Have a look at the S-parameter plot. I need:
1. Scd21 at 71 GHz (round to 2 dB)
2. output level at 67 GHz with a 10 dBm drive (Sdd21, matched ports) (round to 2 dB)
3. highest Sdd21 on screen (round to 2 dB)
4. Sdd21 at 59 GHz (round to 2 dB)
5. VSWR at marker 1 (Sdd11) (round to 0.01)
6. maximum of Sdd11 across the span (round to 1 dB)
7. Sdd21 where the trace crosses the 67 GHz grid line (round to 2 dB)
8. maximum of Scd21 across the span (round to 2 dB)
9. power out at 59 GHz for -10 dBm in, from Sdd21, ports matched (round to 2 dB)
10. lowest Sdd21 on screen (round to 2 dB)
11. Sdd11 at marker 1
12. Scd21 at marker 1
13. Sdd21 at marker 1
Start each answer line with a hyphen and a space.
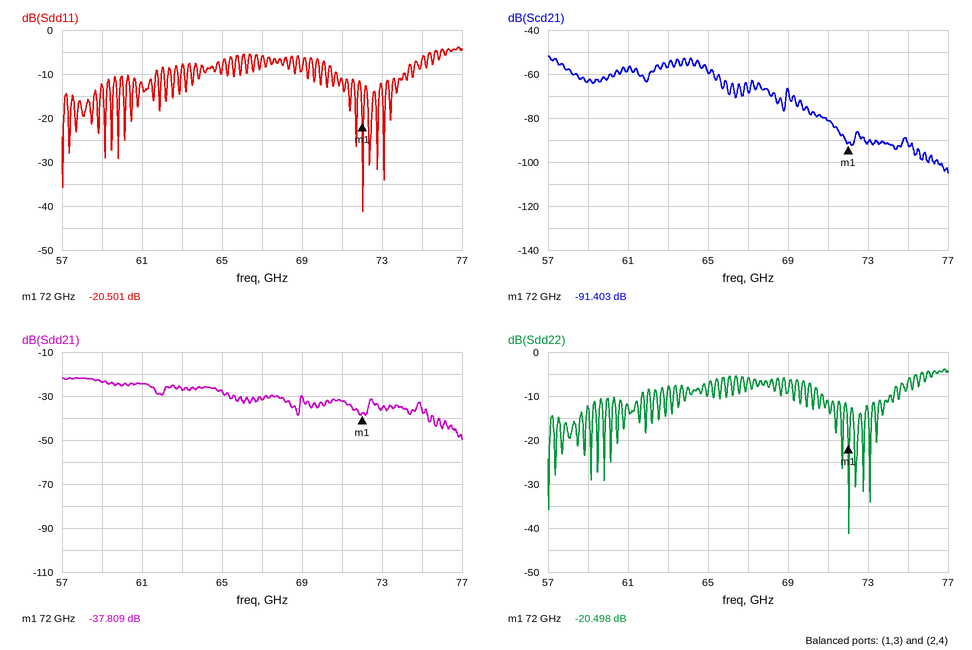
- -82 dB
- -22 dBm
- -22 dB
- -24 dB
- 1.21
- -4 dB
- -32 dB
- -52 dB
- -34 dBm
- -50 dB
- -20.501 dB
- -91.403 dB
- -37.809 dB
